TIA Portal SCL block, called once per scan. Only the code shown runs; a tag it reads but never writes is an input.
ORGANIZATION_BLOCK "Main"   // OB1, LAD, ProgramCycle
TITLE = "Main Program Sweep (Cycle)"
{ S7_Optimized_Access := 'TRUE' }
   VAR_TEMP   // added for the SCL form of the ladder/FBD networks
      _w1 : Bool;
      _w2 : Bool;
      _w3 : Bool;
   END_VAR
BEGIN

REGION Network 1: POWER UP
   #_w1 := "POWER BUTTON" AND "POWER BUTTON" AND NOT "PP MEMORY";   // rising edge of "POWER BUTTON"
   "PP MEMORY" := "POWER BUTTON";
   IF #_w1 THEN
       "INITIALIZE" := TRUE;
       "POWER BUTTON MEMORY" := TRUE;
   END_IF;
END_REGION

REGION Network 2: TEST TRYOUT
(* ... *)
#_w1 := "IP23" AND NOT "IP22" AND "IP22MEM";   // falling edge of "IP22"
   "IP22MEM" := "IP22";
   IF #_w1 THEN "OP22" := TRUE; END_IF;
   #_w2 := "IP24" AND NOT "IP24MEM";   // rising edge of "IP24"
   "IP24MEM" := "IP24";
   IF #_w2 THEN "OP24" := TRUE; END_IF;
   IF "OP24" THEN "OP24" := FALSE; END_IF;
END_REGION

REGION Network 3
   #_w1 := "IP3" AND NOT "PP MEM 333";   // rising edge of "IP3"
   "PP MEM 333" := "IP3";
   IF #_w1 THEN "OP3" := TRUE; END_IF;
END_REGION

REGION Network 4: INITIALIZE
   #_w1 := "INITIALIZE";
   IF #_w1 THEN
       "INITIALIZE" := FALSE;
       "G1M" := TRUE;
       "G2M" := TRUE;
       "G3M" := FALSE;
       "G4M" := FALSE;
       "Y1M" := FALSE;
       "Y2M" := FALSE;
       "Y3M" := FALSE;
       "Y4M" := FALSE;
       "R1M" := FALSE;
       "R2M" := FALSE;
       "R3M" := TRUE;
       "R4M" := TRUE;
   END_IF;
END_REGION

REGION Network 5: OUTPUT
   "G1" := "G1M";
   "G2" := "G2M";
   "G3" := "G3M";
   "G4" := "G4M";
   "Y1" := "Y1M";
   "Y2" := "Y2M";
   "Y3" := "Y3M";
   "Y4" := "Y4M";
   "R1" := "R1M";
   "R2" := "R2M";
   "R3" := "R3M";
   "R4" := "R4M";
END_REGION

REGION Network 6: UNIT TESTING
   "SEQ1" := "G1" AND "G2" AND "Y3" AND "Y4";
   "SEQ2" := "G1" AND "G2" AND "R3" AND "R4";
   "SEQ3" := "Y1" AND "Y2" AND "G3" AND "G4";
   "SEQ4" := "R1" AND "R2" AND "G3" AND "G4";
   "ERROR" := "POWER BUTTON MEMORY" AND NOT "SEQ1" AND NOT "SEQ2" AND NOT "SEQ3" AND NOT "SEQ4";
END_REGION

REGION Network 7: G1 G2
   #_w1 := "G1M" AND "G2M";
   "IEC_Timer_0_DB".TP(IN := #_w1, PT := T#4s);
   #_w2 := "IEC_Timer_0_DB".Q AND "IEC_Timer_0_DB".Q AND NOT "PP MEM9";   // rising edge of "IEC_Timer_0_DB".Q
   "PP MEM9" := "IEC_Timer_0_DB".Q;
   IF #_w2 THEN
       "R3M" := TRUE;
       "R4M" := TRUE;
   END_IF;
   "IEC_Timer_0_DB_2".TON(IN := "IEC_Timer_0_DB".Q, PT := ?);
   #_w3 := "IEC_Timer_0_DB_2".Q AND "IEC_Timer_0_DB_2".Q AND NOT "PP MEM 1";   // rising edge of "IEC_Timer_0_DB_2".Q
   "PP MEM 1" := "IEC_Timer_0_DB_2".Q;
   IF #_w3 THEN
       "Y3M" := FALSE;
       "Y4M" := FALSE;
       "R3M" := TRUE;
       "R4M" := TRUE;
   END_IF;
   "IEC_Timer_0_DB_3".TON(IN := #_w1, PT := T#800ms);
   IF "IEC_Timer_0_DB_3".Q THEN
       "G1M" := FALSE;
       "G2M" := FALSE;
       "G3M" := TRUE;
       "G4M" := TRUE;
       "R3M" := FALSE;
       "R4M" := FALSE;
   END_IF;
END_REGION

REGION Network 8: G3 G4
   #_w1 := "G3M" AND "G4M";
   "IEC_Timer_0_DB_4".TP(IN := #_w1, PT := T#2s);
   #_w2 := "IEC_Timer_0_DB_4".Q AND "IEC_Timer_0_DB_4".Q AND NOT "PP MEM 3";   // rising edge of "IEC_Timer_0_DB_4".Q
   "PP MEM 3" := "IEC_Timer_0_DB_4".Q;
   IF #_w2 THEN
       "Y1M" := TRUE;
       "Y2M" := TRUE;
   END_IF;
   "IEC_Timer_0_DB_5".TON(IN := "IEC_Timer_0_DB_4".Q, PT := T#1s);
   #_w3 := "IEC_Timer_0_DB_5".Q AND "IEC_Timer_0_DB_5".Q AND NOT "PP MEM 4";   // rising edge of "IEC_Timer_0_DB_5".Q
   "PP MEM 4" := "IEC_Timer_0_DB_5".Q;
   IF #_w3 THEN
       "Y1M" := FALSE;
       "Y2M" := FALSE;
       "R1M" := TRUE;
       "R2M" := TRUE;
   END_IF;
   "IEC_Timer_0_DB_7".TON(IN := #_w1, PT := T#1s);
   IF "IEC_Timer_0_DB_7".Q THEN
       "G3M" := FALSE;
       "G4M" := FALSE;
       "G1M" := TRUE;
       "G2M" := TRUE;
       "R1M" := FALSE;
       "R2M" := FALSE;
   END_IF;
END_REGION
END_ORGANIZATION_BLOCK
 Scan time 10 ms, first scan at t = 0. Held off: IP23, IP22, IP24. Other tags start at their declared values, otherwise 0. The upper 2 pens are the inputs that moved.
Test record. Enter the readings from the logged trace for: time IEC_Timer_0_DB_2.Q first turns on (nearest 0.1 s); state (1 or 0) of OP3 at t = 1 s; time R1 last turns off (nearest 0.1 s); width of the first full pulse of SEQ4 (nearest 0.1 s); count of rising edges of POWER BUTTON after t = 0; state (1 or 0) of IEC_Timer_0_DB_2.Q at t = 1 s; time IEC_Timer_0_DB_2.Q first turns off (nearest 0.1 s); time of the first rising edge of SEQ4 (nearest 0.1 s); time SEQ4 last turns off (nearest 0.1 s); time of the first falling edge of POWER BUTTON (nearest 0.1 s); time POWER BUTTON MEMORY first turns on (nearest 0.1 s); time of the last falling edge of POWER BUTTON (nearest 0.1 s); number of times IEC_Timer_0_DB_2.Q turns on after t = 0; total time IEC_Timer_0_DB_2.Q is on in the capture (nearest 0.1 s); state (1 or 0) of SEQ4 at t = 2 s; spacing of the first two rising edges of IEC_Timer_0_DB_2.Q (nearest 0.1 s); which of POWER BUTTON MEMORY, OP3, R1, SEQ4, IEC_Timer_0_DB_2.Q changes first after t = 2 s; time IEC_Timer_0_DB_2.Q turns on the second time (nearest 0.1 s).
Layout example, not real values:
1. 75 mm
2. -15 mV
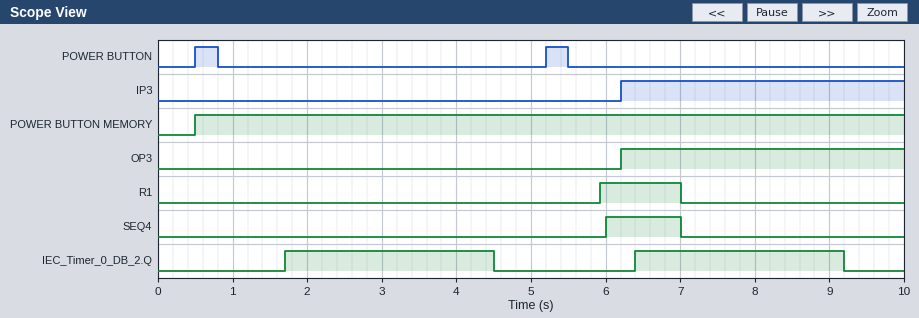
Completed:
1. 1.7 s
2. 0
3. 7.0 s
4. 1.0 s
5. 2
6. 0
7. 4.5 s
8. 6.0 s
9. 7.0 s
10. 0.8 s
11. 0.5 s
12. 5.5 s
13. 2
14. 5.6 s
15. 0
16. 4.7 s
17. IEC_Timer_0_DB_2.Q
18. 6.4 s
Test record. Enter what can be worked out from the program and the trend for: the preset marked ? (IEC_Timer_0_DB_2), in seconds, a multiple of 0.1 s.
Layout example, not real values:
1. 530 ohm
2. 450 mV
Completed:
1. 1.2 s
